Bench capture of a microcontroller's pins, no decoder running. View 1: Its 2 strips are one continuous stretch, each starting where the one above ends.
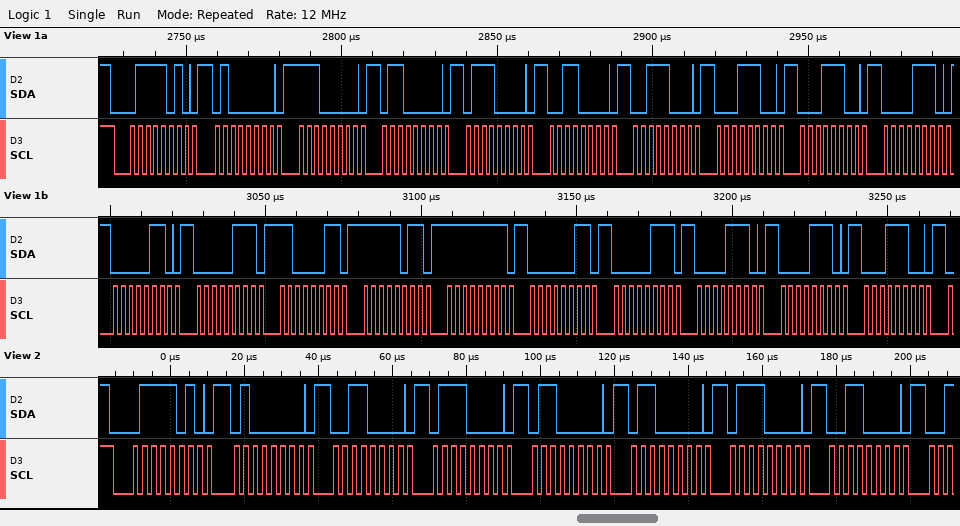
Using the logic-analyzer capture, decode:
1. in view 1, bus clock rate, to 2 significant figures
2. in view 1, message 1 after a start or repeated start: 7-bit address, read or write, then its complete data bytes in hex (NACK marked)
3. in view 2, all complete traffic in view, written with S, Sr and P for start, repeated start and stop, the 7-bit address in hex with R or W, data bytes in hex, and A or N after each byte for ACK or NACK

400 kHz
0x3D write: 40 E0 60 70 30 38 1C 1C 0E 06 07 C3 FB FF 03 07 0E 0E 1C
S 3DW A 40 A 30 A 70 A 60 A 60 A 70 A 30 A
